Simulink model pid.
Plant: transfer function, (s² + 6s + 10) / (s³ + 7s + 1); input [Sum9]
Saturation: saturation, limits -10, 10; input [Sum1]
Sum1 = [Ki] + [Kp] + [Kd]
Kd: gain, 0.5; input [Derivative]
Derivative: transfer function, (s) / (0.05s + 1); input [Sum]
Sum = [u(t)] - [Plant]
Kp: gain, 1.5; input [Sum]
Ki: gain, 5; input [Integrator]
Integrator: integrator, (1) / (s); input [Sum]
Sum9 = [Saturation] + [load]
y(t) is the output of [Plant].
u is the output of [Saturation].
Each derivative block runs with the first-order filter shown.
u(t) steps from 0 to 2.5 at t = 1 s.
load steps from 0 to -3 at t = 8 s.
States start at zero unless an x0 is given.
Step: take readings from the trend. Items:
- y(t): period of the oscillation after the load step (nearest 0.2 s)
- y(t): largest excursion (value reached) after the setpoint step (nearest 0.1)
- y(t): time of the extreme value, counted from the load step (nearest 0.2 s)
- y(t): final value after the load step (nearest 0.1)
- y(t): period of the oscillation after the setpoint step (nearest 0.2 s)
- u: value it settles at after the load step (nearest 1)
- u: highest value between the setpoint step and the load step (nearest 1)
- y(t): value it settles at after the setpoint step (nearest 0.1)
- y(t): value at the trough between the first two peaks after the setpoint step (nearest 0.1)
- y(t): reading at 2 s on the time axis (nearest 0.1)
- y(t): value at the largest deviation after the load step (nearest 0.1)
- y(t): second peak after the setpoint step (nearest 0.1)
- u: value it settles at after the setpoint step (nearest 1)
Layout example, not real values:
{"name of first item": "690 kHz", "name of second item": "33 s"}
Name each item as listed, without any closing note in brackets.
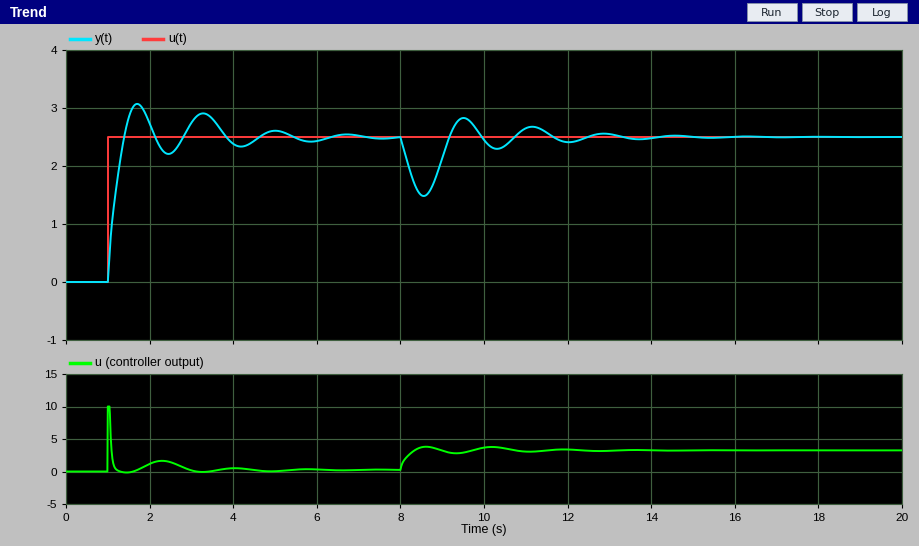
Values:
{"y(t): period of the oscillation after the load step": "1.8 s", "y(t): largest excursion (value reached) after the setpoint step": "3.1", "y(t): time of the extreme value, counted from the load step": "0.6 s", "y(t): final value after the load step": "2.5", "y(t): period of the oscillation after the setpoint step": "1.6 s", "u: value it settles at after the load step": "3", "u: highest value between the setpoint step and the load step": "10", "y(t): value it settles at after the setpoint step": "2.5", "y(t): value at the trough between the first two peaks after the setpoint step": "2.2", "y(t): reading at 2 s on the time axis": "2.7", "y(t): value at the largest deviation after the load step": "1.5", "y(t): second peak after the setpoint step": "2.9", "u: value it settles at after the setpoint step": "0"}
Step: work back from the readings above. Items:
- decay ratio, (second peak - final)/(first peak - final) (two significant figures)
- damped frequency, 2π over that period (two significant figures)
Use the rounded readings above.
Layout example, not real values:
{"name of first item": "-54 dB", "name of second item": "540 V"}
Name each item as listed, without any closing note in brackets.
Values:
{"decay ratio, (second peak - final)/(first peak - final)": "0.67", "damped frequency, 2π over that period": "3.9 rad/s"}
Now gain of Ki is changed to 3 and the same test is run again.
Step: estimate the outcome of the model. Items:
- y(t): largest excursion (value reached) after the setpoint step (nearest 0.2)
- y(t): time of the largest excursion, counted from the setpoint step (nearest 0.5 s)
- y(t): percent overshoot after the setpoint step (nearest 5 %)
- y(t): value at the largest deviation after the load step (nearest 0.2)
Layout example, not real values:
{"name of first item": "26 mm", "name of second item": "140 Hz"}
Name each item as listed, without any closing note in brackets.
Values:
{"y(t): largest excursion (value reached) after the setpoint step": "2.8", "y(t): time of the largest excursion, counted from the setpoint step": "2.5 s", "y(t): percent overshoot after the setpoint step": "15 %", "y(t): value at the largest deviation after the load step": "1.4"}
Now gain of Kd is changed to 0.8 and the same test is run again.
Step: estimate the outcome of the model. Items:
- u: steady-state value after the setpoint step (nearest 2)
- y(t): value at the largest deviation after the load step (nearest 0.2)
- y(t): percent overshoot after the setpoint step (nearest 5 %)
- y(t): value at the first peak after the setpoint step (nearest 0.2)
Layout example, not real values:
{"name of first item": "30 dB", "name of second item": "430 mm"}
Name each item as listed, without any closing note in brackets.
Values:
{"u: steady-state value after the setpoint step": "0", "y(t): value at the largest deviation after the load step": "1.6", "y(t): percent overshoot after the setpoint step": "15 %", "y(t): value at the first peak after the setpoint step": "2.8"}
